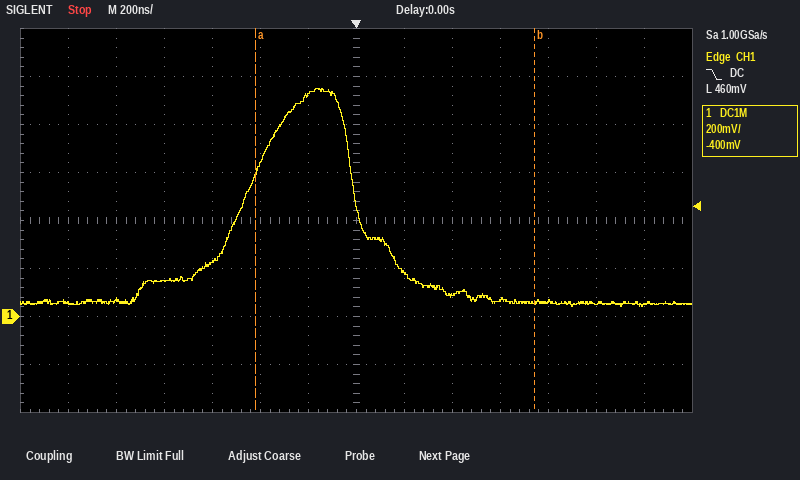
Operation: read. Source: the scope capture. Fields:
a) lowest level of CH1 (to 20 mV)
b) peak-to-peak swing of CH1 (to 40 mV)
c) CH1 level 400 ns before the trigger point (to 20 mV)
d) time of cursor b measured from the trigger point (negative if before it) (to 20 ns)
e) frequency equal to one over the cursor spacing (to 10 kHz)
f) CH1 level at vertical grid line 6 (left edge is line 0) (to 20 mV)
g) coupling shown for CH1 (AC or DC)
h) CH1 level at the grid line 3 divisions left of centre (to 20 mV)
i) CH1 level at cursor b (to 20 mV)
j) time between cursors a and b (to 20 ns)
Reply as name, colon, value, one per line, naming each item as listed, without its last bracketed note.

lowest level of CH1: 40 mV
peak-to-peak swing of CH1: 920 mV
CH1 level 400 ns before the trigger point: 640 mV
time of cursor b measured from the trigger point (negative if before it): +740 ns
frequency equal to one over the cursor spacing: 860 kHz
CH1 level at vertical grid line 6 (left edge is line 0): 920 mV
coupling shown for CH1: DC
CH1 level at the grid line 3 divisions left of centre: 220 mV
CH1 level at cursor b: 60 mV
time between cursors a and b: 1.16 µs
